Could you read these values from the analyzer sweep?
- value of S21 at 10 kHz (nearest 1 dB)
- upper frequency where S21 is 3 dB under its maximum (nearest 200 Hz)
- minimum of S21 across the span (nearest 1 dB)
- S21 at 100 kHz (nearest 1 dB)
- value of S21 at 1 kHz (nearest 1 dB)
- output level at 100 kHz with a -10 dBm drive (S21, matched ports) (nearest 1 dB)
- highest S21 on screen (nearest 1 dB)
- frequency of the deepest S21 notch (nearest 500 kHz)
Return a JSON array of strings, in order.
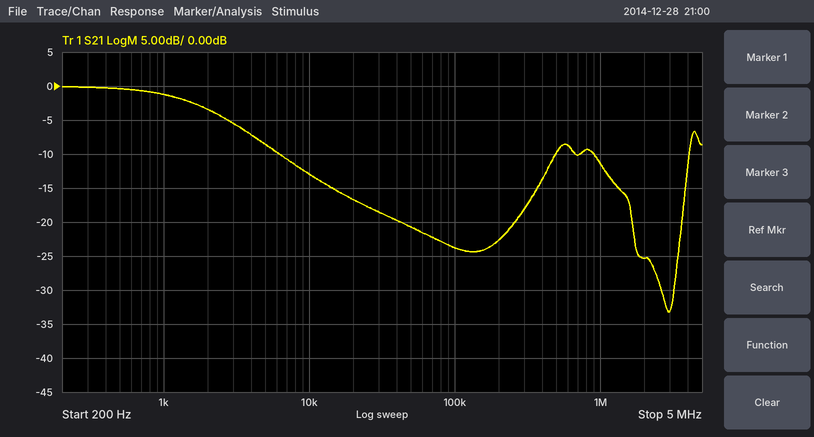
["-13 dB", "1.8 kHz", "-33 dB", "-24 dB", "-1 dB", "-34 dBm", "0 dB", "3.0 MHz"]
